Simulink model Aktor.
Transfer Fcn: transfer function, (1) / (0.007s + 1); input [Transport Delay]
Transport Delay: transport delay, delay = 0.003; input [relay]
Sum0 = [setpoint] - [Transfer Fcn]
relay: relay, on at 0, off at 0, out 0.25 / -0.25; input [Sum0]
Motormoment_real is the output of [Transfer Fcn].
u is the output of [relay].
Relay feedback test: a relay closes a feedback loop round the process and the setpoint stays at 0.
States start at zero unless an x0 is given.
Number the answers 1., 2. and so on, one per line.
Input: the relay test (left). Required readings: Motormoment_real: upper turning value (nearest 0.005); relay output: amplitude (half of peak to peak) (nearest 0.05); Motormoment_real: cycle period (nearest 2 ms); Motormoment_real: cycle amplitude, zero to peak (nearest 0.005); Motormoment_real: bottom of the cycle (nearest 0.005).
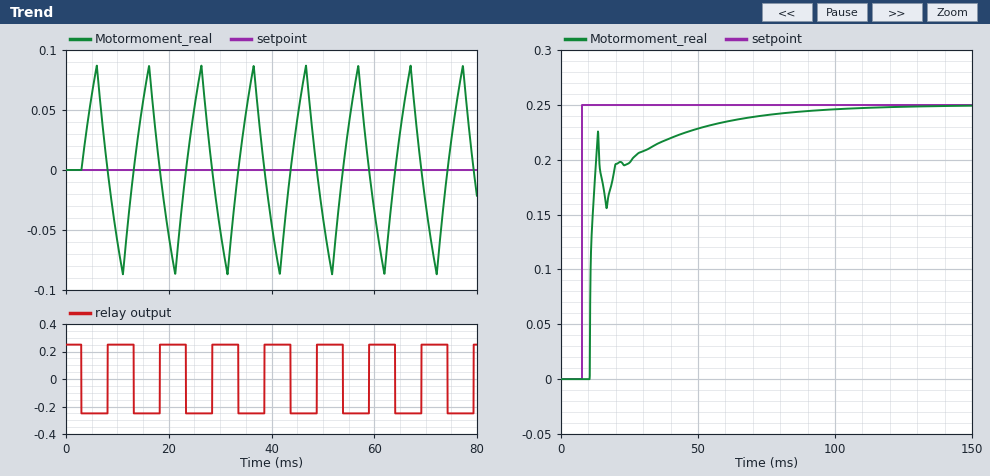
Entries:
1. 0.085
2. 0.25
3. 10 ms
4. 0.085
5. -0.085
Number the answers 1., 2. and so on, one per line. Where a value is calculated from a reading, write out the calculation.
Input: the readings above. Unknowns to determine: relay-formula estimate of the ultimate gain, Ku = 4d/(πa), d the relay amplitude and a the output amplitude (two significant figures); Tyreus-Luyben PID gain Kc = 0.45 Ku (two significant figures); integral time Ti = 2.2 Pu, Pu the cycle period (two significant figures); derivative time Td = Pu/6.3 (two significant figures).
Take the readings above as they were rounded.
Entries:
1. 4 × 0.25 / (π × 0.085) = 3.7
2. 0.45 × 3.7 = 1.7
3. 2.2 × 10 = 22 ms
4. 10 / 6.3 = 1.6 ms
